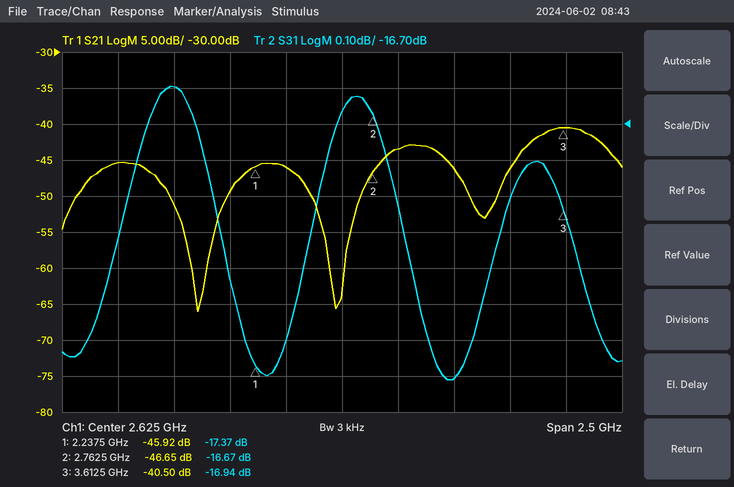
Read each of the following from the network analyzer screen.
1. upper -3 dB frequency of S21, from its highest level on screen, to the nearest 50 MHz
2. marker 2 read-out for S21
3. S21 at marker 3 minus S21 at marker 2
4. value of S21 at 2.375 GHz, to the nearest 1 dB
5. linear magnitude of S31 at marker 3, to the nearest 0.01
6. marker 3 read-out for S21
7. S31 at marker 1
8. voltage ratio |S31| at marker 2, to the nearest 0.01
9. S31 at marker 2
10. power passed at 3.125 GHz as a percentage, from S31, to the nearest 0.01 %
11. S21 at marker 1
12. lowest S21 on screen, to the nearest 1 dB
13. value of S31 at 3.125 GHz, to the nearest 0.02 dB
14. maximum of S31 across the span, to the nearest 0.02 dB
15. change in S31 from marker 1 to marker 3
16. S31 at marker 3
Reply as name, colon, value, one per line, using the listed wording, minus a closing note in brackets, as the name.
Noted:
upper -3 dB frequency of S21, from its highest level on screen, to the nearest 50 MHz: 3.80 GHz
marker 2 read-out for S21: -46.65 dB
S21 at marker 3 minus S21 at marker 2: 6.15 dB
value of S21 at 2.375 GHz, to the nearest 1 dB: -46 dB
linear magnitude of S31 at marker 3, to the nearest 0.01: 0.14
marker 3 read-out for S21: -40.50 dB
S31 at marker 1: -17.37 dB
voltage ratio |S31| at marker 2, to the nearest 0.01: 0.15
S31 at marker 2: -16.67 dB
power passed at 3.125 GHz as a percentage, from S31, to the nearest 0.01 %: 1.82 %
S21 at marker 1: -45.92 dB
lowest S21 on screen, to the nearest 1 dB: -66 dB
value of S31 at 3.125 GHz, to the nearest 0.02 dB: -17.40 dB
maximum of S31 across the span, to the nearest 0.02 dB: -16.60 dB
change in S31 from marker 1 to marker 3: 0.43 dB
S31 at marker 3: -16.94 dB
